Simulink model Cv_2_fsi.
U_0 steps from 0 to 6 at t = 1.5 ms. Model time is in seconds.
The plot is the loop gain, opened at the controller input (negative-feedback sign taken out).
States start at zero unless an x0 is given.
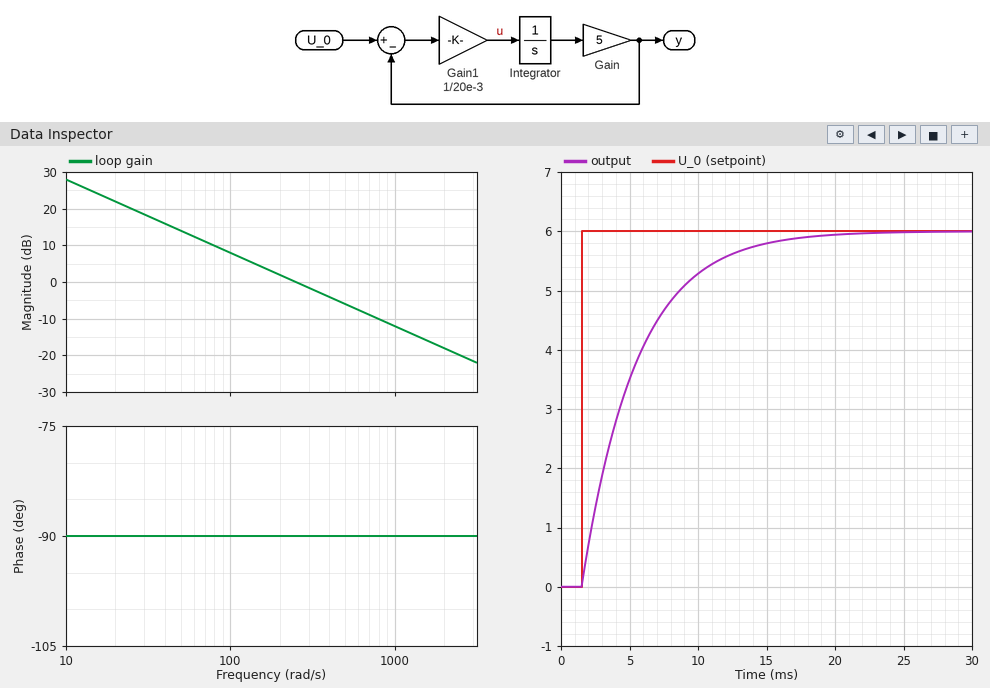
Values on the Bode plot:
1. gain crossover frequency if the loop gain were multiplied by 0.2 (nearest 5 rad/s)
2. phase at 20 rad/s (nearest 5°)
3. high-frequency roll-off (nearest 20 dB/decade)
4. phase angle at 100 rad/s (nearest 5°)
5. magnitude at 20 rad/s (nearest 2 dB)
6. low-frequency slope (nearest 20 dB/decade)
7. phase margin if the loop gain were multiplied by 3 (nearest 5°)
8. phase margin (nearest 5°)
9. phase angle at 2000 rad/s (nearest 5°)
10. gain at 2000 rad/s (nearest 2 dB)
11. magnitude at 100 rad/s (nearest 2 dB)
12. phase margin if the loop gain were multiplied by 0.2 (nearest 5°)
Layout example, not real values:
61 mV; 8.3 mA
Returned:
50 rad/s; -90°; -20 dB/decade; -90°; 22 dB; -20 dB/decade; 90°; 90°; -90°; -18 dB; 8 dB; 90°
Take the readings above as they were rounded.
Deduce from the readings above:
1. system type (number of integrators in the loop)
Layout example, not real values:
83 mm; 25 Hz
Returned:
1
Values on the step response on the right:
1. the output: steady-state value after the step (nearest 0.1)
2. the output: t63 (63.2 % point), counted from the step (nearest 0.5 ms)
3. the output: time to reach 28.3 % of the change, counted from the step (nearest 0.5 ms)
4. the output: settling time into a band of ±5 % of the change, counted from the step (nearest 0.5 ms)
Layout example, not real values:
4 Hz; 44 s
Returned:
6.0; 4.0 ms; 1.5 ms; 12.0 ms
